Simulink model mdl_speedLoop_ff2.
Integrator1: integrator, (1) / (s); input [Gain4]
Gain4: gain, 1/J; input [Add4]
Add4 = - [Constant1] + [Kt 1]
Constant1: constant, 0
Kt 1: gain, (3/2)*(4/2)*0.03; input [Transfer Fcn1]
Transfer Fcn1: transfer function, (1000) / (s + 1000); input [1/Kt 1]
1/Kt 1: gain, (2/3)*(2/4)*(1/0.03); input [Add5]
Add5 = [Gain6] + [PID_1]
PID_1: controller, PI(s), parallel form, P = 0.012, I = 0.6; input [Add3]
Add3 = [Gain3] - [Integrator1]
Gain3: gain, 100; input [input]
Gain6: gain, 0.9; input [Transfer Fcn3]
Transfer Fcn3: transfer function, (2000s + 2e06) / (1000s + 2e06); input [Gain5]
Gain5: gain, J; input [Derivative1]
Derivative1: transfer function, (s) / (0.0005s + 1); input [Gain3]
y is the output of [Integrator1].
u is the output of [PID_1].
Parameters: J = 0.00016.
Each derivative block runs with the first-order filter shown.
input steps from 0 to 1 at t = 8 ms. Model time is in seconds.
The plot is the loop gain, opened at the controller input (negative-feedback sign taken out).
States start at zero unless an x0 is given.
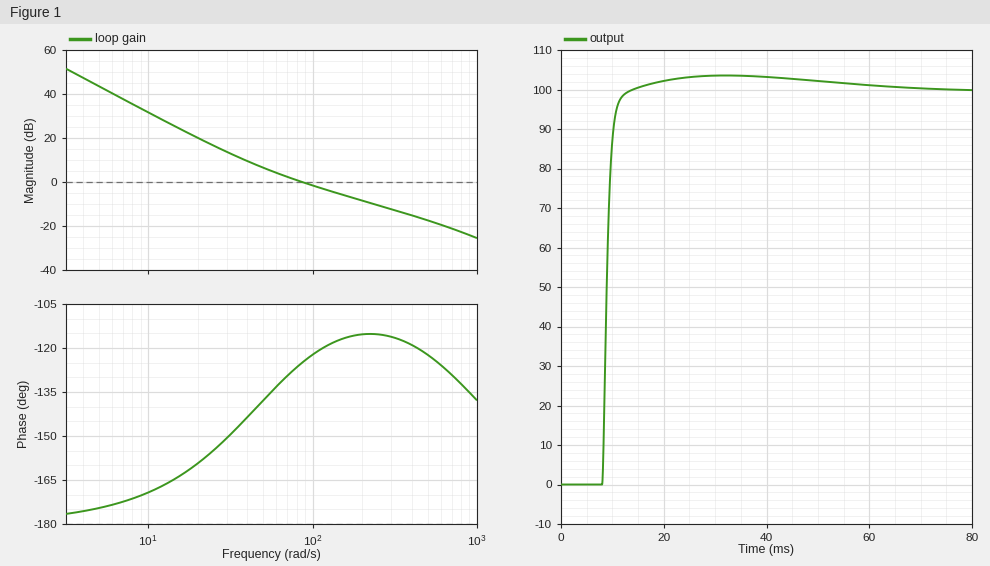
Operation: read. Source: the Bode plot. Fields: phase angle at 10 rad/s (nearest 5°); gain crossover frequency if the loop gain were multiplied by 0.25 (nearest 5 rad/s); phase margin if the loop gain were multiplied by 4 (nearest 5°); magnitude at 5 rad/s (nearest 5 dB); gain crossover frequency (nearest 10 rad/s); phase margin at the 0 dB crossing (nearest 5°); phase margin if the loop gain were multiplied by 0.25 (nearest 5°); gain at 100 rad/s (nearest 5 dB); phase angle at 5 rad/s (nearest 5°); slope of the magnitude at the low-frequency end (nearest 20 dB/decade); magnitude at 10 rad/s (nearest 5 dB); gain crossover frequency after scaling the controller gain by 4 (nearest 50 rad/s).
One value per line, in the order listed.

-170°
35 rad/s
65°
45 dB
90 rad/s
55°
30°
0 dB
-175°
-40 dB/decade
30 dB
300 rad/s
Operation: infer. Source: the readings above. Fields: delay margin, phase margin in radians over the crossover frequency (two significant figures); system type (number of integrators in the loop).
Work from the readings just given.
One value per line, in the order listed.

0.011 s
2
